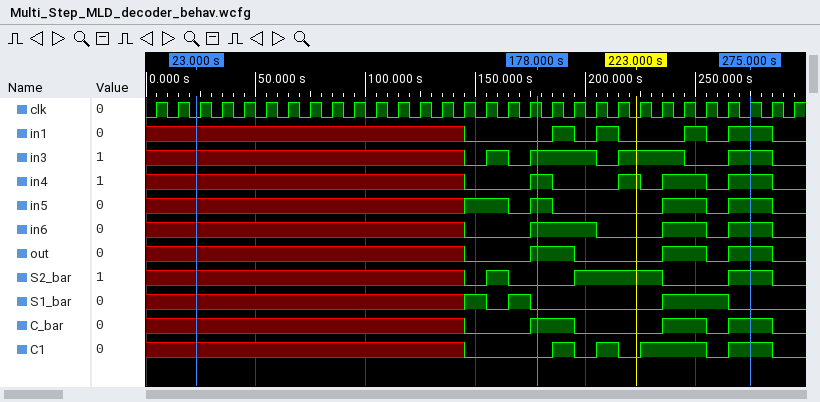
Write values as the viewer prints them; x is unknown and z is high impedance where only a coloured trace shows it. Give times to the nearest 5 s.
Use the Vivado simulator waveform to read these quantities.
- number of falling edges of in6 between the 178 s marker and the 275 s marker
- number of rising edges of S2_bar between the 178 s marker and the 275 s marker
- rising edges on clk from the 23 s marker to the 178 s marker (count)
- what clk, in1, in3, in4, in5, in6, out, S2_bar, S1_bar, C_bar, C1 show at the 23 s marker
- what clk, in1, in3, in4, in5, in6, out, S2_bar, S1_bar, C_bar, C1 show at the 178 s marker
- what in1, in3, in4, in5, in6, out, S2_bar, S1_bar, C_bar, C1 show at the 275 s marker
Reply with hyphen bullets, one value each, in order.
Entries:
- 2
- 2
- 16
- clk=0, in1=x, in3=x, in4=x, in5=x, in6=x, out=x, S2_bar=x, S1_bar=x, C_bar=x, C1=x
- clk=1, in1=0, in3=1, in4=1, in5=1, in6=1, out=1, S2_bar=0, S1_bar=0, C_bar=1, C1=0
- in1=1, in3=1, in4=1, in5=1, in6=1, out=1, S2_bar=1, S1_bar=0, C_bar=1, C1=1
